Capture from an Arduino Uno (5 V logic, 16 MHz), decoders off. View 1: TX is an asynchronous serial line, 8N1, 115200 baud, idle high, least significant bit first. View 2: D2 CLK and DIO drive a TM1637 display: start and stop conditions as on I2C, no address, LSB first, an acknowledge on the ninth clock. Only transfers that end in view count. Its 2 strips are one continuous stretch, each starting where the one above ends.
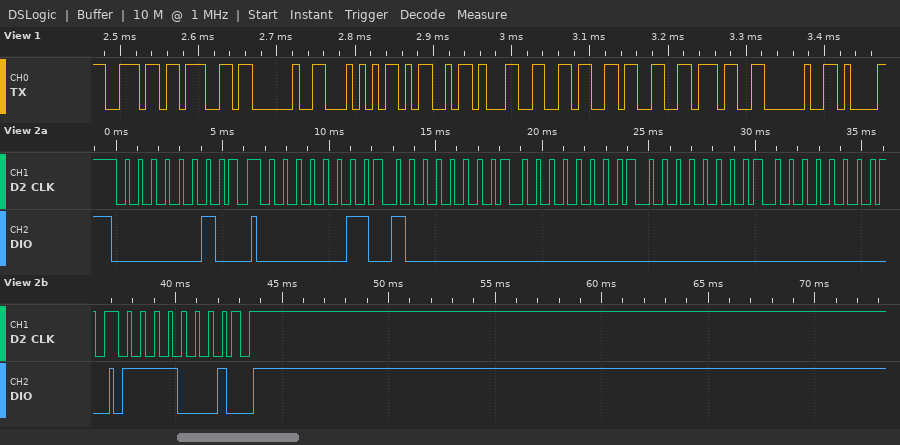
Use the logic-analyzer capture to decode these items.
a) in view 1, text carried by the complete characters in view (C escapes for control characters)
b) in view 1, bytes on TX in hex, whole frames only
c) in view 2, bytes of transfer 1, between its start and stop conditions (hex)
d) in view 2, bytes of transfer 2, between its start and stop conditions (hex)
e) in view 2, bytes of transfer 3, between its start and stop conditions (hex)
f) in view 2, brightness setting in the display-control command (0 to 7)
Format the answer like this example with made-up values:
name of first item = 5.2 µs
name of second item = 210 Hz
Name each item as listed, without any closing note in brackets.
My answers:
in view 1, text carried by the complete characters in view = "ng TM1637 "
in view 1, bytes on TX in hex, whole frames only = 6E 67 20 54 4D 31 36 33 37 20
in view 2, bytes of transfer 1, between its start and stop conditions = 40
in view 2, bytes of transfer 2, between its start and stop conditions = C0 01 00 00 00
in view 2, bytes of transfer 3, between its start and stop conditions = 8F
in view 2, brightness setting in the display-control command = 7
